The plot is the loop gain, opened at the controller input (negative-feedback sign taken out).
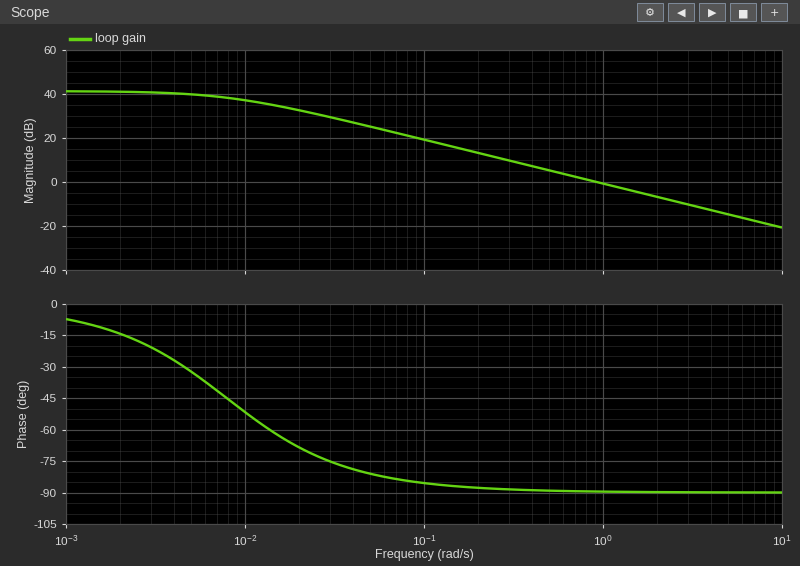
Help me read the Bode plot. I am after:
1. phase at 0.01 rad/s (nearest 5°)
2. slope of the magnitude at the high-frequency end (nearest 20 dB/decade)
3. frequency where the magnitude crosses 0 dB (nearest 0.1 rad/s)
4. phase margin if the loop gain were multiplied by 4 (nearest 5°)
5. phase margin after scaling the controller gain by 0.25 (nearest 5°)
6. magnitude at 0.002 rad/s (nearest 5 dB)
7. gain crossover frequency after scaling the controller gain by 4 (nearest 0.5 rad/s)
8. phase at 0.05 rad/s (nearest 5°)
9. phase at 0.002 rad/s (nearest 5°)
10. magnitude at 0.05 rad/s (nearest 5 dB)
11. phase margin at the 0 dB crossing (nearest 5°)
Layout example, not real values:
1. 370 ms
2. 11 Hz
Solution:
1. -50°
2. -20 dB/decade
3. 0.9 rad/s
4. 90°
5. 90°
6. 40 dB
7. 3.5 rad/s
8. -80°
9. -15°
10. 25 dB
11. 90°
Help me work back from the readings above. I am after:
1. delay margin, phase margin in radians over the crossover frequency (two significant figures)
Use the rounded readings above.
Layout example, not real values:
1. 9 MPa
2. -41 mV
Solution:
1. 1.7 s
